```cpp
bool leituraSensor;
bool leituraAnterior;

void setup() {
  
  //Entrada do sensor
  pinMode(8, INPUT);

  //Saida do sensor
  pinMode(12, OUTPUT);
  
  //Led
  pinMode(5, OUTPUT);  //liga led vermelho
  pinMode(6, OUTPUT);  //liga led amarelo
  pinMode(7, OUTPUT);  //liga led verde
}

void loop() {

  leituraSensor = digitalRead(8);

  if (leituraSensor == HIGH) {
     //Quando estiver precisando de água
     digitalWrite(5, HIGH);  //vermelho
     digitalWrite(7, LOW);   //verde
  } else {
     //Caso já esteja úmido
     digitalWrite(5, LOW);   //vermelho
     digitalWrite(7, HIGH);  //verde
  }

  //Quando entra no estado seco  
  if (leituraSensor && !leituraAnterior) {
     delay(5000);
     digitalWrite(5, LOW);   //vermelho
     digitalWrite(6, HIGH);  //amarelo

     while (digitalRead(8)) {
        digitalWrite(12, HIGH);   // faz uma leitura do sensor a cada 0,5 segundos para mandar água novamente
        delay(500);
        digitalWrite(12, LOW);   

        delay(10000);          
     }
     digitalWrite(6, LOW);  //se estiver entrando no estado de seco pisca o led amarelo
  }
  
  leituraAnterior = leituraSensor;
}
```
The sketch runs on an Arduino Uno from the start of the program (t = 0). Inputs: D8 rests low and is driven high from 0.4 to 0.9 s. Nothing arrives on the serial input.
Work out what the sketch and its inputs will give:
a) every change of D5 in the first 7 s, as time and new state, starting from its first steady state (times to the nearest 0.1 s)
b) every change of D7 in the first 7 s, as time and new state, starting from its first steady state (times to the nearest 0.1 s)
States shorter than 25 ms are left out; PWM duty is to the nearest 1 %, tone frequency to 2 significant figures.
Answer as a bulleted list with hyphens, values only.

- 0 s low; 0.4 s high; 5.4 s low
- 0 s high; 0.4 s low; 5.4 s high
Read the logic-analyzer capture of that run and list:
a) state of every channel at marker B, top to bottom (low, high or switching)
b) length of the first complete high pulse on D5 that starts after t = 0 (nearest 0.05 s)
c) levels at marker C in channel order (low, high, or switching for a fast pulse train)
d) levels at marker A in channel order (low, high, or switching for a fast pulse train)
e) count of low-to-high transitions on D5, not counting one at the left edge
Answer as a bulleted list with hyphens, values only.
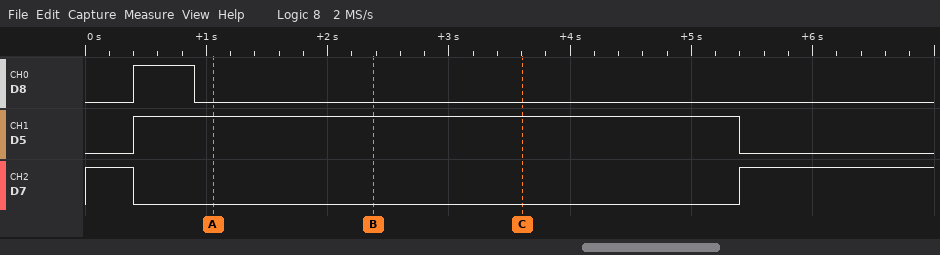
- D8 low, D5 high, D7 low
- 5.00 s
- D8 low, D5 high, D7 low
- D8 low, D5 high, D7 low
- 1
